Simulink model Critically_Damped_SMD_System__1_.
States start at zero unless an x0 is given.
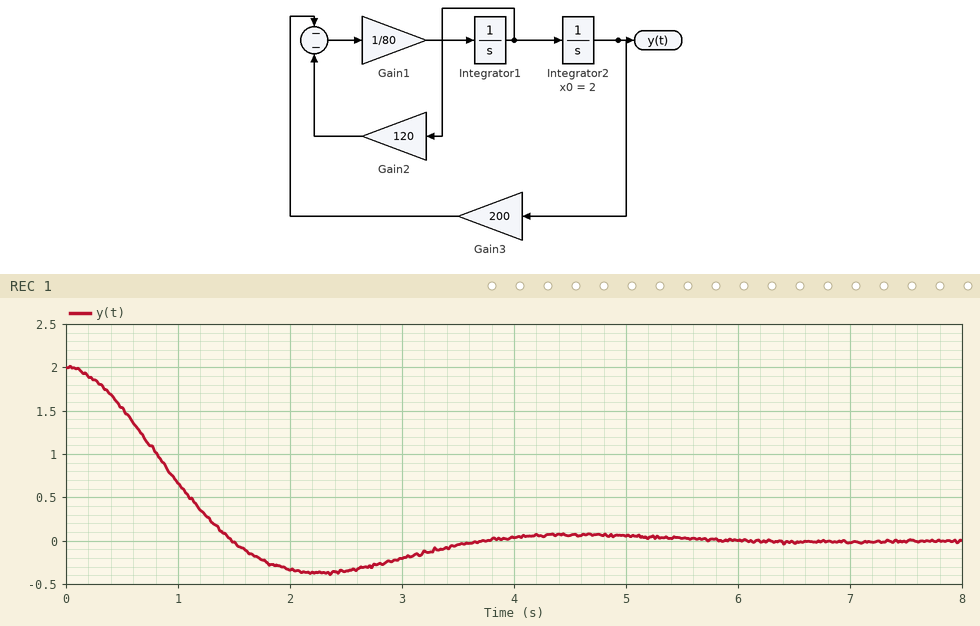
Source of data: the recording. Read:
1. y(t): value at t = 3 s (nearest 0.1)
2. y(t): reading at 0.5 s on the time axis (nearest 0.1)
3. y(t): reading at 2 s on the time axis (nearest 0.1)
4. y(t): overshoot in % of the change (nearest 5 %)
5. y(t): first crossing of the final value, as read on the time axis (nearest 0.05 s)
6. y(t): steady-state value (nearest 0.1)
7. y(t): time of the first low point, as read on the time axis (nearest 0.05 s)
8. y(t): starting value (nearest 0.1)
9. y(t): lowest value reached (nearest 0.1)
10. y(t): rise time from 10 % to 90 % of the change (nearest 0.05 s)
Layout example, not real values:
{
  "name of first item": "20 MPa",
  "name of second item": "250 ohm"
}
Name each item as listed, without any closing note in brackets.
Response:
{
  "y(t): value at t = 3 s": "-0.2",
  "y(t): reading at 0.5 s on the time axis": "1.5",
  "y(t): reading at 2 s on the time axis": "-0.3",
  "y(t): overshoot in % of the change": "20 %",
  "y(t): first crossing of the final value, as read on the time axis": "1.50 s",
  "y(t): steady-state value": "0.0",
  "y(t): time of the first low point, as read on the time axis": "2.25 s",
  "y(t): starting value": "2.0",
  "y(t): lowest value reached": "-0.4",
  "y(t): rise time from 10 % to 90 % of the change": "1.00 s"
}
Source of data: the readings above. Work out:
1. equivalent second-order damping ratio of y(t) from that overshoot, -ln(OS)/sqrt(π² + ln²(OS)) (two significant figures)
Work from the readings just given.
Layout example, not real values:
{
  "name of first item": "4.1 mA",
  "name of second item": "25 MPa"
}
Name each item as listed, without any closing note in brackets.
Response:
{
  "equivalent second-order damping ratio of y(t) from that overshoot, -ln(OS)/sqrt(π² + ln²(OS))": "0.46"
}
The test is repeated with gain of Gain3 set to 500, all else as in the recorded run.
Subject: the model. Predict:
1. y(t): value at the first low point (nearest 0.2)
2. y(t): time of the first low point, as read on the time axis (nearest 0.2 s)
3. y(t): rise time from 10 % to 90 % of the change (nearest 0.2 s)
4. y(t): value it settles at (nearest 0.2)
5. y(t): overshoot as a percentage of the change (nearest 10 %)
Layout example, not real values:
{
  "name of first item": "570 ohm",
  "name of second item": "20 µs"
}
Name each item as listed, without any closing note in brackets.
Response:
{
  "y(t): value at the first low point": "-0.8",
  "y(t): time of the first low point, as read on the time axis": "1.4 s",
  "y(t): rise time from 10 % to 90 % of the change": "0.6 s",
  "y(t): value it settles at": "0.0",
  "y(t): overshoot as a percentage of the change": "40 %"
}
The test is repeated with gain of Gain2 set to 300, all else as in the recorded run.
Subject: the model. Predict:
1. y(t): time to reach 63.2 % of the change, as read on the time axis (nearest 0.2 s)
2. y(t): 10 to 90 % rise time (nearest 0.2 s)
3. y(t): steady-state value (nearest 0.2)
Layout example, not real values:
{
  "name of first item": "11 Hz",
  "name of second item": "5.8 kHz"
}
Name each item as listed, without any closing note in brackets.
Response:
{
  "y(t): time to reach 63.2 % of the change, as read on the time axis": "1.6 s",
  "y(t): 10 to 90 % rise time": "2.8 s",
  "y(t): steady-state value": "0.0"
}
